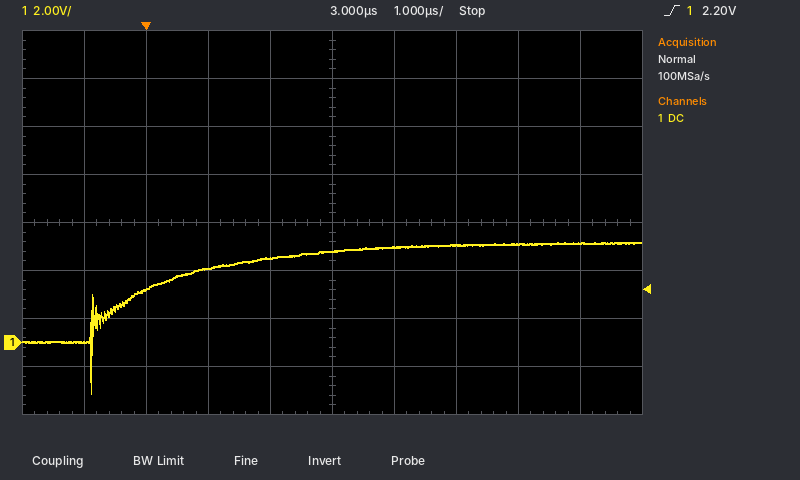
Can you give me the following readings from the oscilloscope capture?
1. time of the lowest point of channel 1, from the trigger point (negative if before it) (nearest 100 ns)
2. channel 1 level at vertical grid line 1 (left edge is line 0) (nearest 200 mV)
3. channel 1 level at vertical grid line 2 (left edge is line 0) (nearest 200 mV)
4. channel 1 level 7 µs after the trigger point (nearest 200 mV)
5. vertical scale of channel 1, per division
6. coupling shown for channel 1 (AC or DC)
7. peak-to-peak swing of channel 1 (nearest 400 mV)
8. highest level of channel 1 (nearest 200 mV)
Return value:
-900 ns
0.0 V
2.2 V
4.2 V
2 V
DC
6.4 V
4.2 V
